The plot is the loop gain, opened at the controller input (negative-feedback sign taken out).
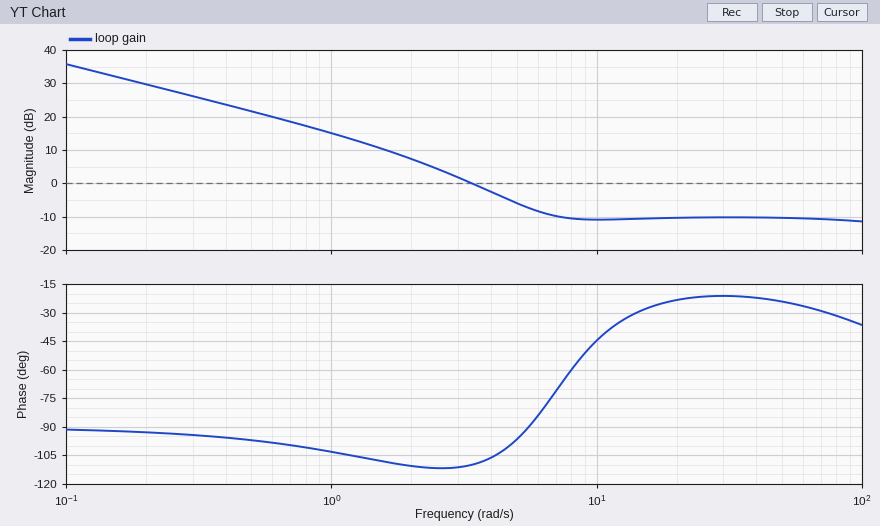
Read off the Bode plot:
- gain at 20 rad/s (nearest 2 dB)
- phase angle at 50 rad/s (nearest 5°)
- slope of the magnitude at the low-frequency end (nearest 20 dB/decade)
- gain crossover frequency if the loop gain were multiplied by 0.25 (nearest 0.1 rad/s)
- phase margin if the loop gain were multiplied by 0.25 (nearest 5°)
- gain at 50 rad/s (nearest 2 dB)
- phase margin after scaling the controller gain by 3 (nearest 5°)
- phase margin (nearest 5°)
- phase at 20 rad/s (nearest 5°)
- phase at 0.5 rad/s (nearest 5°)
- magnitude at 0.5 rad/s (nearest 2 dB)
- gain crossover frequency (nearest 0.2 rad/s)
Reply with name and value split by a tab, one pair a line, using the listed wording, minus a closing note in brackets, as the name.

gain at 20 rad/s	-10 dB
phase angle at 50 rad/s	-25°
slope of the magnitude at the low-frequency end	-20 dB/decade
gain crossover frequency if the loop gain were multiplied by 0.25	1.3 rad/s
phase margin if the loop gain were multiplied by 0.25	75°
gain at 50 rad/s	-10 dB
phase margin after scaling the controller gain by 3	105°
phase margin	70°
phase at 20 rad/s	-25°
phase at 0.5 rad/s	-95°
magnitude at 0.5 rad/s	22 dB
gain crossover frequency	3.4 rad/s
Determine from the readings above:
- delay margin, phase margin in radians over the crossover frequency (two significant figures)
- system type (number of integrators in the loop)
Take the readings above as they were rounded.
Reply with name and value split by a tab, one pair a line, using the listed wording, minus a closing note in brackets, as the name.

delay margin, phase margin in radians over the crossover frequency	0.36 s
system type	1
